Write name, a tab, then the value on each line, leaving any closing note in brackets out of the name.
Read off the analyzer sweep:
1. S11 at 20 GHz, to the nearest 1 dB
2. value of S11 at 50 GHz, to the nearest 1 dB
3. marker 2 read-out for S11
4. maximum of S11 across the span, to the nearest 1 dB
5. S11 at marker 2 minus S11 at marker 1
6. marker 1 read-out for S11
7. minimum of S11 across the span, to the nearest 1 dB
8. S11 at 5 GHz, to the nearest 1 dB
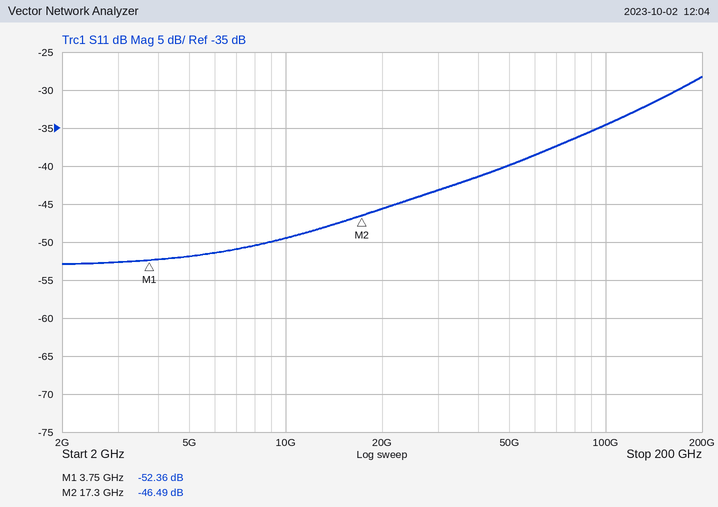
S11 at 20 GHz, to the nearest 1 dB	-46 dB
value of S11 at 50 GHz, to the nearest 1 dB	-40 dB
marker 2 read-out for S11	-46.49 dB
maximum of S11 across the span, to the nearest 1 dB	-28 dB
S11 at marker 2 minus S11 at marker 1	5.87 dB
marker 1 read-out for S11	-52.36 dB
minimum of S11 across the span, to the nearest 1 dB	-53 dB
S11 at 5 GHz, to the nearest 1 dB	-52 dB
